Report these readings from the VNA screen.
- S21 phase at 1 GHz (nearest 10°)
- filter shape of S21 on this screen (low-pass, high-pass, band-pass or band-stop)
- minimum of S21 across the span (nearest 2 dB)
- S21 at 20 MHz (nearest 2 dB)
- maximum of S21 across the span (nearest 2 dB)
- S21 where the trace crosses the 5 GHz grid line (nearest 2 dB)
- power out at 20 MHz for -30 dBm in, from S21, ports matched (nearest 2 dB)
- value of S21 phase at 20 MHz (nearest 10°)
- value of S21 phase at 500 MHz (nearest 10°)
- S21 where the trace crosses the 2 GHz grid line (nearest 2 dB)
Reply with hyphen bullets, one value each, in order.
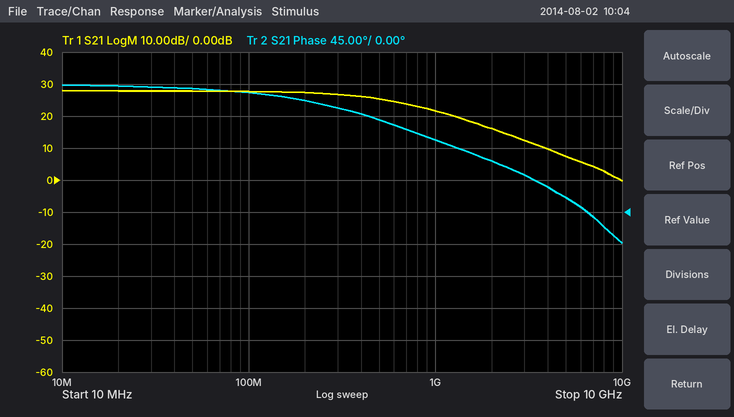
- 100°
- low-pass
- 0 dB
- 28 dB
- 28 dB
- 8 dB
- -2 dBm
- 180°
- 130°
- 16 dB
